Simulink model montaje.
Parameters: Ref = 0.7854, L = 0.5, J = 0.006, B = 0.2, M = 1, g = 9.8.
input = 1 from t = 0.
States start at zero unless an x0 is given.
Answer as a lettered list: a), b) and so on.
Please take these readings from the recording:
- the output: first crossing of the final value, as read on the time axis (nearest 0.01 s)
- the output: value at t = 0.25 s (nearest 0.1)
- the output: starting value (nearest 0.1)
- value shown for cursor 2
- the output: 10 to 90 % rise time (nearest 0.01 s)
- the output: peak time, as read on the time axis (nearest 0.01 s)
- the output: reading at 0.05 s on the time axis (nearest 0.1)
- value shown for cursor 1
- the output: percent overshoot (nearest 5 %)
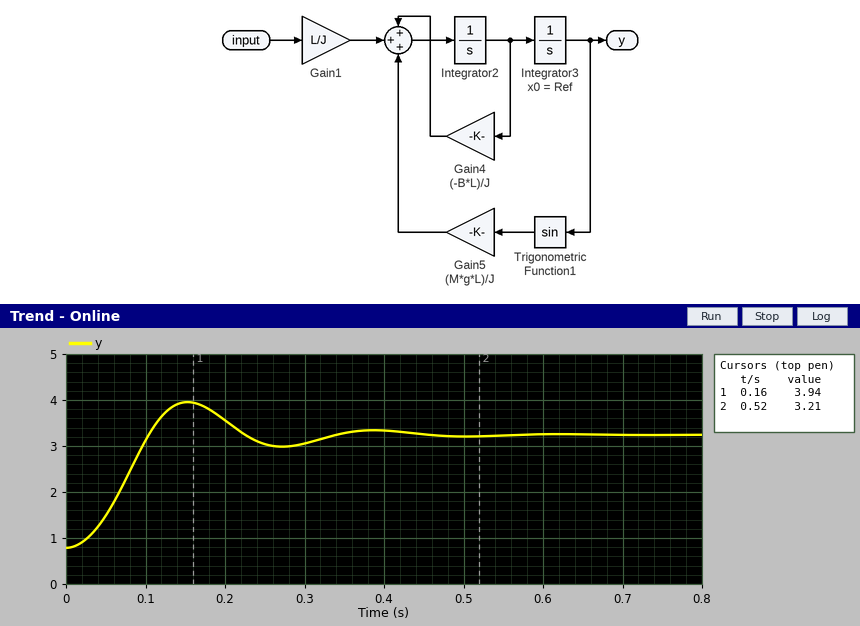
a) 0.10 s
b) 3.0
c) 0.8
d) 3.21
e) 0.07 s
f) 0.15 s
g) 1.5
h) 3.94
i) 30 %
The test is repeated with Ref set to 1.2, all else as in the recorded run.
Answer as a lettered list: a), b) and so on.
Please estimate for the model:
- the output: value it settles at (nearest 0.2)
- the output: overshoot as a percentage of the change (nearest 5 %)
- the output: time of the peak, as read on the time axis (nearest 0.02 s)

a) 3.2
b) 30 %
c) 0.14 s
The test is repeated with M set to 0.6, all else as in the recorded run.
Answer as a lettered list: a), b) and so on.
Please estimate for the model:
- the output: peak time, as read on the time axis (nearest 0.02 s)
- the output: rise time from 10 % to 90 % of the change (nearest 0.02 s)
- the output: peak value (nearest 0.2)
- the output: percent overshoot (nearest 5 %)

a) 0.20 s
b) 0.10 s
c) 3.8
d) 20 %
